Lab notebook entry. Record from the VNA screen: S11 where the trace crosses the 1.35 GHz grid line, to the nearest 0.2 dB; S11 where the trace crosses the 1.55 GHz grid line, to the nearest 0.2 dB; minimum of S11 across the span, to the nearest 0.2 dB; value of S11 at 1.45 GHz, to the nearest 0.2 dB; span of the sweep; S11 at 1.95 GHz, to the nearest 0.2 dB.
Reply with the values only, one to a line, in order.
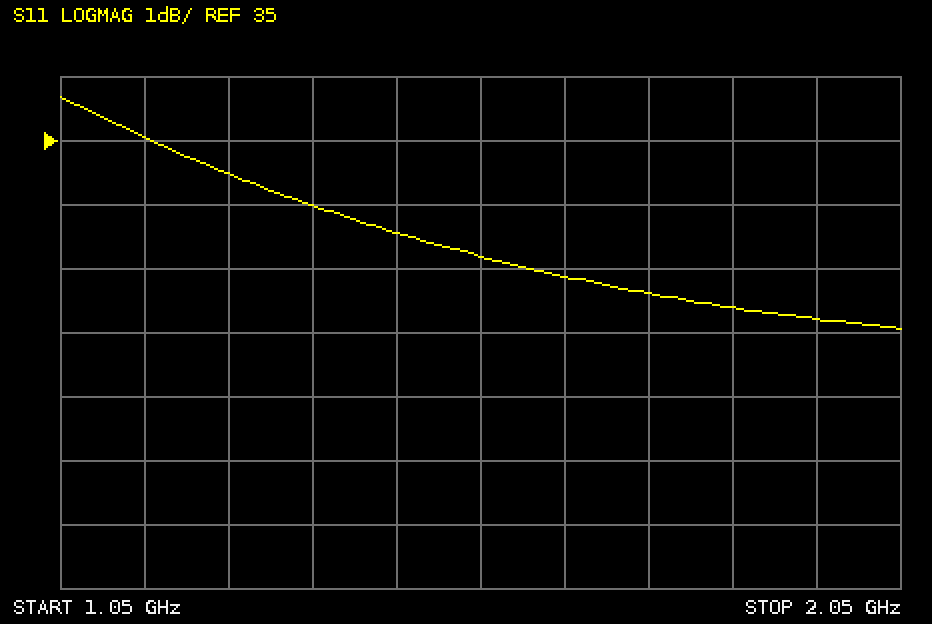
34.0 dB
33.2 dB
32.0 dB
33.6 dB
1 GHz
32.2 dB
